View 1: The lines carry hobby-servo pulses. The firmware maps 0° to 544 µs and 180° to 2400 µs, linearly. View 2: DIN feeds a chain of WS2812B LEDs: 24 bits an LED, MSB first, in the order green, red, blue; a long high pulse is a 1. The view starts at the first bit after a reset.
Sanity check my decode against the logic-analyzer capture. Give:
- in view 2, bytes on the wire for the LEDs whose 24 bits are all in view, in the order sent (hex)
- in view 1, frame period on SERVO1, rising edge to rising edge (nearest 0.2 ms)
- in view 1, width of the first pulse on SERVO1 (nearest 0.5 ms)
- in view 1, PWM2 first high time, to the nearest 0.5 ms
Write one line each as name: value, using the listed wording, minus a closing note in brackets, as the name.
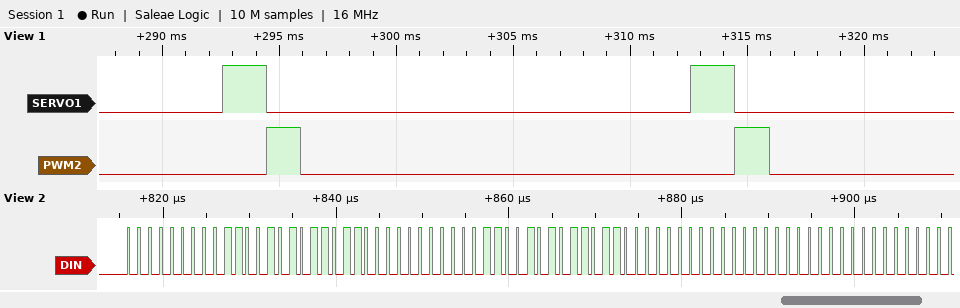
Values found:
in view 2, bytes on the wire for the LEDs whose 24 bits are all in view, in the order sent: 00 65 6C 00 65 6C 00 00 00
in view 1, frame period on SERVO1, rising edge to rising edge: 20.0 ms
in view 1, width of the first pulse on SERVO1: 2.0 ms
in view 1, PWM2 first high time, to the nearest 0.5 ms: 1.5 ms
